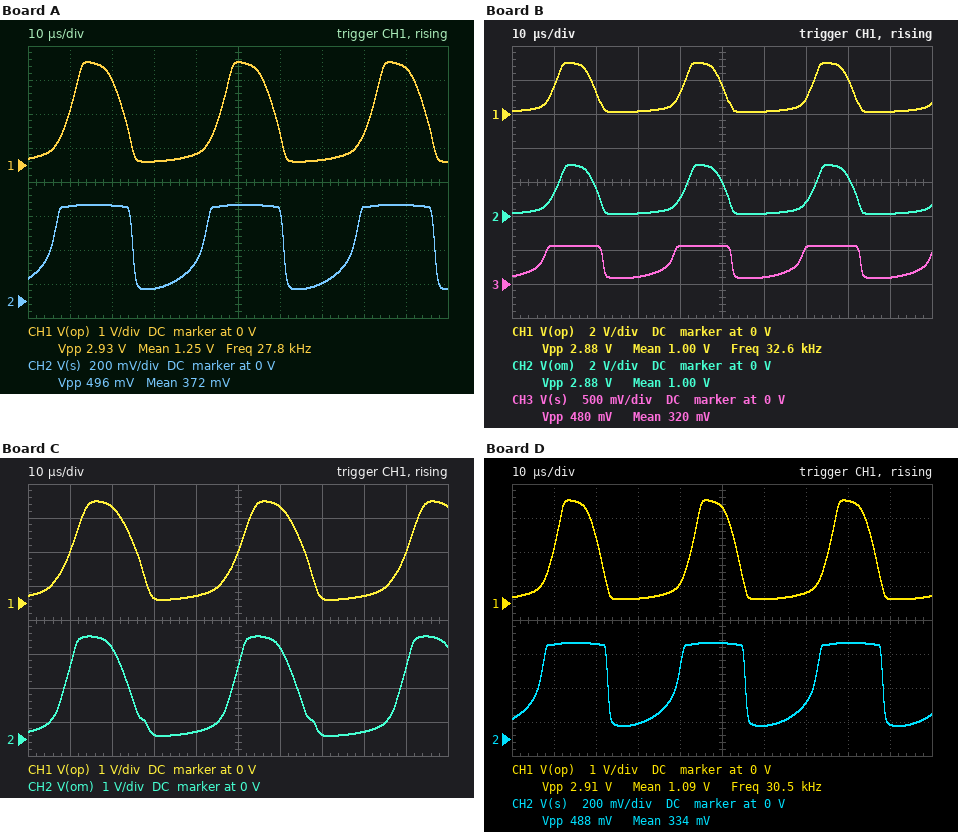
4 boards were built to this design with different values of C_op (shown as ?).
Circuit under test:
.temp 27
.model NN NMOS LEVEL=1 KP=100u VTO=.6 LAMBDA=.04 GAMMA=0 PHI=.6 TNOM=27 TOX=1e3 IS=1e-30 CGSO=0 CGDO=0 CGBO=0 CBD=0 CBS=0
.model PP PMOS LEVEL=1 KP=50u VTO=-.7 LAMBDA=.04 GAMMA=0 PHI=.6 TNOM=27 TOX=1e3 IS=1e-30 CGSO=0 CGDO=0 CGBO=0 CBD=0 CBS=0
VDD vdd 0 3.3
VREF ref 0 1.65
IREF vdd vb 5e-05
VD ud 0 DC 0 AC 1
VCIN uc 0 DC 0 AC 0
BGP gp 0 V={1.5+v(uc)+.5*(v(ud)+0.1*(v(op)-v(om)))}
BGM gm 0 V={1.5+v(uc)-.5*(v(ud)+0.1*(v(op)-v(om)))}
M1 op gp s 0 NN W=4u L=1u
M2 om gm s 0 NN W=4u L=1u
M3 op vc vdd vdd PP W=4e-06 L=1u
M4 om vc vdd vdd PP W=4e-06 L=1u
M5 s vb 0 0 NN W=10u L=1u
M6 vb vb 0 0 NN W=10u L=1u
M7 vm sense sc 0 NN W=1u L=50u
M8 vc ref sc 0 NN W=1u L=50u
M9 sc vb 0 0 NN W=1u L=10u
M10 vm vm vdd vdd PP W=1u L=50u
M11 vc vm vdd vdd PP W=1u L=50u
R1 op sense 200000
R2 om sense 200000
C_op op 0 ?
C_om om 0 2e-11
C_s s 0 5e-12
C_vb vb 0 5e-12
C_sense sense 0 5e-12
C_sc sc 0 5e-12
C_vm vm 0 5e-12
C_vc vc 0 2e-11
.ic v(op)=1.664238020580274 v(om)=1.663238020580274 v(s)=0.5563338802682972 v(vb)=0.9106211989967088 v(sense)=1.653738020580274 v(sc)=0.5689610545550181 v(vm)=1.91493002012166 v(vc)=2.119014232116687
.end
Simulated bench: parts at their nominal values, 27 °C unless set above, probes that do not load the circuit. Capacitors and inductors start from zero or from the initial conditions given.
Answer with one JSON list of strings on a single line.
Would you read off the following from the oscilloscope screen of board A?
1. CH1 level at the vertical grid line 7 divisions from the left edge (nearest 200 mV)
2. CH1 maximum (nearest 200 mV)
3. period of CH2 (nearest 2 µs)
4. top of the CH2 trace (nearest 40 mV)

["200 mV", "3.0 V", "36 µs", "560 mV"]
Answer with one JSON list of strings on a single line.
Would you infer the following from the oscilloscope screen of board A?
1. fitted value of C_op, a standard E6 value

["33 pF"]
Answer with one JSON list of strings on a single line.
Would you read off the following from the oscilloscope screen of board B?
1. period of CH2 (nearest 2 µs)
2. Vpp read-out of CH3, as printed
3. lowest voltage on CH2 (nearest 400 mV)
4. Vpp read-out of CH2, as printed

["30 µs", "480 mV", "0 V", "2.88 V"]
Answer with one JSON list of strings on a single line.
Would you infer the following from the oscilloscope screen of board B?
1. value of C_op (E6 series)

["6.8 pF"]
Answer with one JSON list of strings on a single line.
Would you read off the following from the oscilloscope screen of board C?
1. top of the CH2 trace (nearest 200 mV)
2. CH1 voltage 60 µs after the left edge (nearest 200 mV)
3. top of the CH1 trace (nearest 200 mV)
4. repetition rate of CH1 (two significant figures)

["3.0 V", "2.8 V", "3.0 V", "25 kHz"]
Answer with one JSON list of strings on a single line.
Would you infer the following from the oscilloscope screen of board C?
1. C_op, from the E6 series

["68 pF"]
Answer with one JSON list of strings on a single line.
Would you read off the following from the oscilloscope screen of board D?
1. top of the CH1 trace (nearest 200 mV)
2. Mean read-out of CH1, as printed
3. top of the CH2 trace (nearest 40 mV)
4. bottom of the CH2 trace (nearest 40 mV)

["3.0 V", "1.09 V", "560 mV", "80 mV"]
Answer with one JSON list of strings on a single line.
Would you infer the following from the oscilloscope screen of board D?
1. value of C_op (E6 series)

["15 pF"]
